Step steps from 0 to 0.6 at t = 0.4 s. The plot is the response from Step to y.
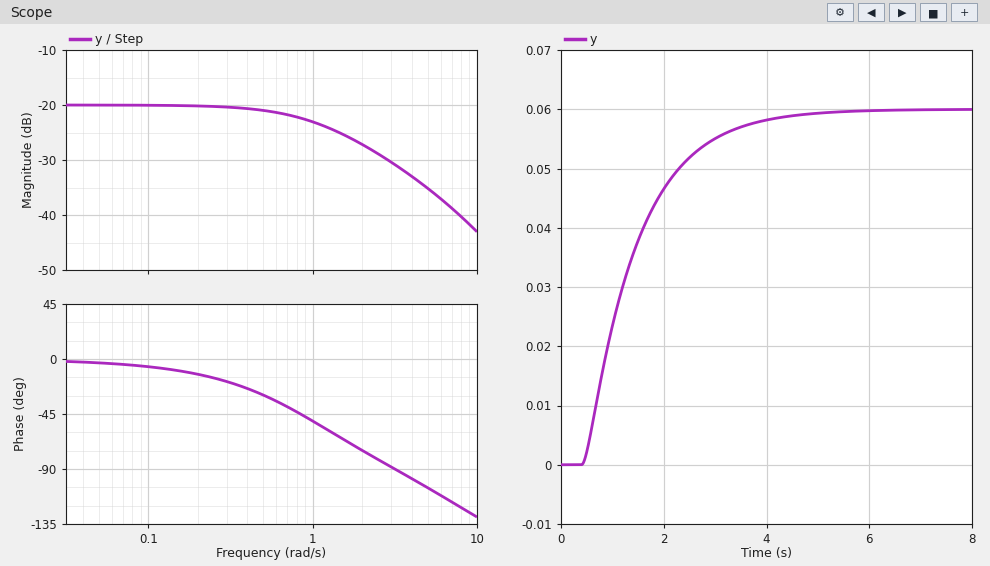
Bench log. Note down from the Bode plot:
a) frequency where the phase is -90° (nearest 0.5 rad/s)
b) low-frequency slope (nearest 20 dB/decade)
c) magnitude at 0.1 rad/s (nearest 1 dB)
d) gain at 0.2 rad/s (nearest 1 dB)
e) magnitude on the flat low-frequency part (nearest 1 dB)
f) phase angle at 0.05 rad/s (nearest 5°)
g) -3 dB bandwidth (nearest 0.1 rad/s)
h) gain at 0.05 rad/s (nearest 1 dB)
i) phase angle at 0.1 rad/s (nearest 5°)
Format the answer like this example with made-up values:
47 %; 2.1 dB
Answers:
3.0 rad/s; 0 dB/decade; -20 dB; -20 dB; -20 dB; -5°; 1.0 rad/s; -20 dB; -5°
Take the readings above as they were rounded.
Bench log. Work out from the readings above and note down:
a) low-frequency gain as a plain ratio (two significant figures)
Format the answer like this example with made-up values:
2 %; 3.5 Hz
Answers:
0.10
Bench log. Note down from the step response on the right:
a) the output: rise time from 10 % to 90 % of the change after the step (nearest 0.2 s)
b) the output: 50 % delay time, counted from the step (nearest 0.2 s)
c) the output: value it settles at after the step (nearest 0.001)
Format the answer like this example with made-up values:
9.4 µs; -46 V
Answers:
2.2 s; 0.8 s; 0.060
